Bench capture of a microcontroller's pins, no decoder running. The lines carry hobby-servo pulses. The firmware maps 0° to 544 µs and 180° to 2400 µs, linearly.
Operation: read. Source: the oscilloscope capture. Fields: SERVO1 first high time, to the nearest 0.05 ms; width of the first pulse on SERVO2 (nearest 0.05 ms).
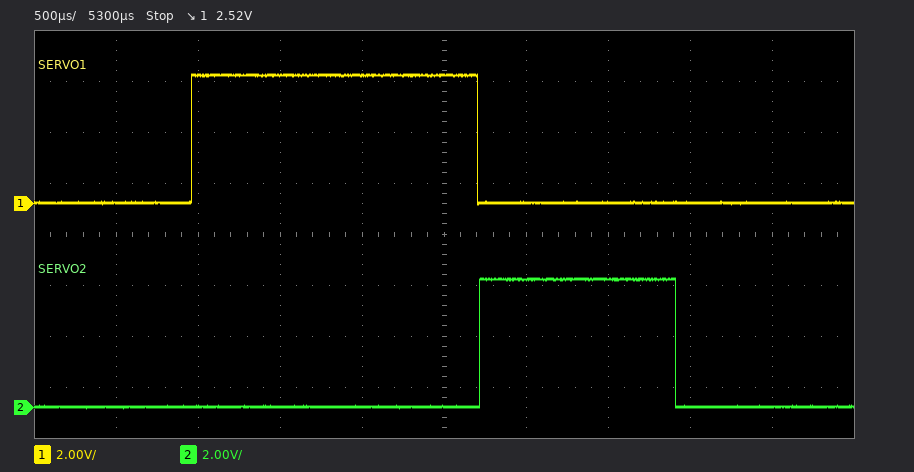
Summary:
1.75 ms
1.20 ms
